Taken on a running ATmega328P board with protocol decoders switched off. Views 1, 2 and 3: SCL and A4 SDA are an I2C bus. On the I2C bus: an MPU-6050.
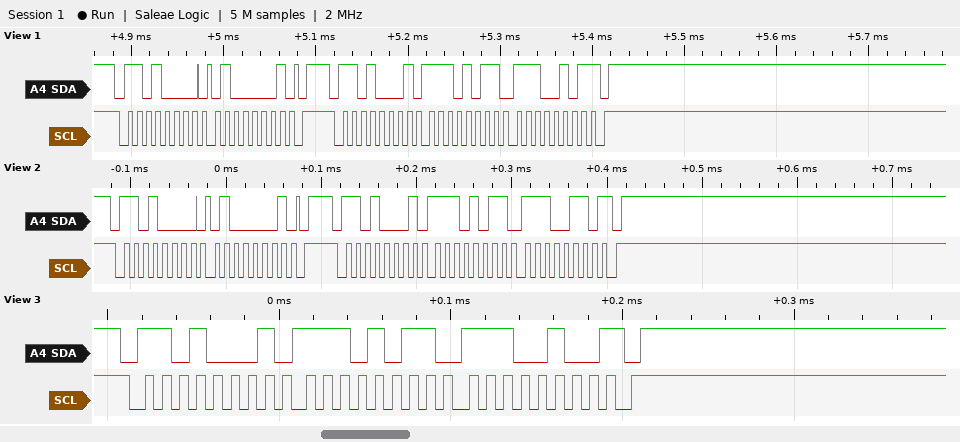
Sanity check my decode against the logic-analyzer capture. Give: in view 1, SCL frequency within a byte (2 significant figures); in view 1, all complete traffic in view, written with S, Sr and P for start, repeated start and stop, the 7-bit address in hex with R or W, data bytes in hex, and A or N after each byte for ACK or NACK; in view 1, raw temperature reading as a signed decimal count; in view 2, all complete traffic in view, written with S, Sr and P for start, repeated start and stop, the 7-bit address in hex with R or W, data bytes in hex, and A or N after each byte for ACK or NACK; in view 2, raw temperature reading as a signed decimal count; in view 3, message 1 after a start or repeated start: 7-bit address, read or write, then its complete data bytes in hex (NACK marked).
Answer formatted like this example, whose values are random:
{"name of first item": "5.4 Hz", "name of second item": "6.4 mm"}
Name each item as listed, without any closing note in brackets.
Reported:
{"in view 1, SCL frequency within a byte": "100 kHz", "in view 1, all complete traffic in view, written with S, Sr and P for start, repeated start and stop, the 7-bit address in hex with R or W, data bytes in hex, and A or N after each byte for ACK or NACK": "S 68W A 41 A P S 68R A EB A E5 N P", "in view 1, raw temperature reading as a signed decimal count": "-5147", "in view 2, all complete traffic in view, written with S, Sr and P for start, repeated start and stop, the 7-bit address in hex with R or W, data bytes in hex, and A or N after each byte for ACK or NACK": "S 68W A 41 A P S 68R A EB A E6 N P", "in view 2, raw temperature reading as a signed decimal count": "-5146", "in view 3, message 1 after a start or repeated start: 7-bit address, read or write, then its complete data bytes in hex": "0x68 read: EB E4 NACK"}
